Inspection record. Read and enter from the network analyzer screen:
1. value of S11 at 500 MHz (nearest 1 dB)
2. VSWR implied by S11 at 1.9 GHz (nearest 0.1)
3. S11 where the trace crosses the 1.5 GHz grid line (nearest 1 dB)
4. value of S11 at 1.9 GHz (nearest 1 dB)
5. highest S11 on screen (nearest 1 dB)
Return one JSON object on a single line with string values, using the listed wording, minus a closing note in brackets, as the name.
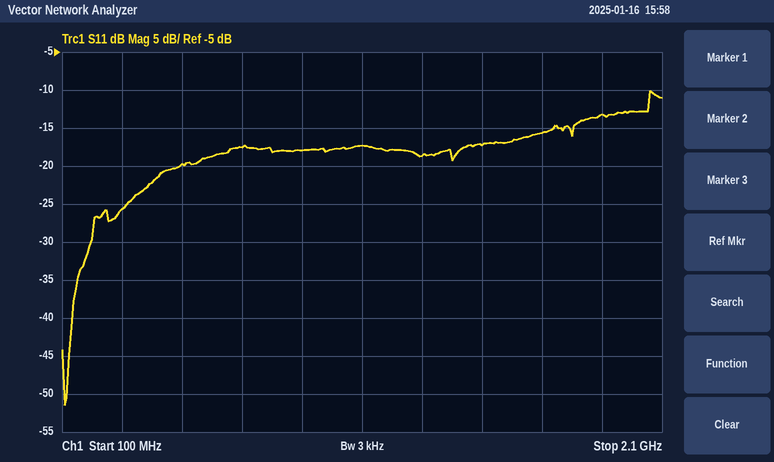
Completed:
{"value of S11 at 500 MHz": "-20 dB", "VSWR implied by S11 at 1.9 GHz": "1.6", "S11 where the trace crosses the 1.5 GHz grid line": "-17 dB", "value of S11 at 1.9 GHz": "-13 dB", "highest S11 on screen": "-10 dB"}
